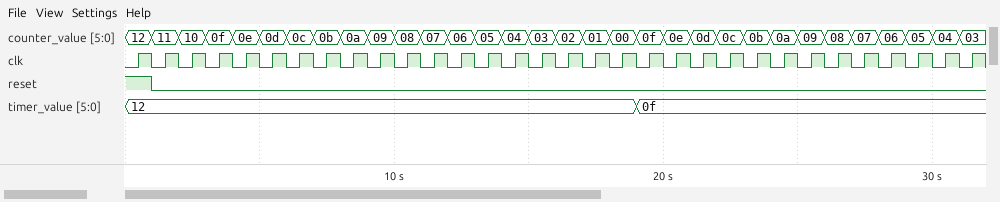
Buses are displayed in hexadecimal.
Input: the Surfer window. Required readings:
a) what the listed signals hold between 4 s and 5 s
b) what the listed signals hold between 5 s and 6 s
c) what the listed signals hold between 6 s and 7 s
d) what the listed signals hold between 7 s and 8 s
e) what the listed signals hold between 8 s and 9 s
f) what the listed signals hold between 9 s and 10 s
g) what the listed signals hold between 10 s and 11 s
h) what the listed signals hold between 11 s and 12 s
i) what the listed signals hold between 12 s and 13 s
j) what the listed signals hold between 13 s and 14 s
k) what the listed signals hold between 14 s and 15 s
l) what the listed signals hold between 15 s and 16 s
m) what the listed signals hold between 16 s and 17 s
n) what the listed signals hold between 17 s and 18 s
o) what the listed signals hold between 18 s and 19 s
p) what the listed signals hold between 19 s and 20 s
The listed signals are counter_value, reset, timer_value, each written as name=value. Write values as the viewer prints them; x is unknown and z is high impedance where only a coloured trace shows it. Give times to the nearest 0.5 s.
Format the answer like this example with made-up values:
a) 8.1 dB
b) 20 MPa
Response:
a) counter_value=0e, reset=0, timer_value=12
b) counter_value=0d, reset=0, timer_value=12
c) counter_value=0c, reset=0, timer_value=12
d) counter_value=0b, reset=0, timer_value=12
e) counter_value=0a, reset=0, timer_value=12
f) counter_value=09, reset=0, timer_value=12
g) counter_value=08, reset=0, timer_value=12
h) counter_value=07, reset=0, timer_value=12
i) counter_value=06, reset=0, timer_value=12
j) counter_value=05, reset=0, timer_value=12
k) counter_value=04, reset=0, timer_value=12
l) counter_value=03, reset=0, timer_value=12
m) counter_value=02, reset=0, timer_value=12
n) counter_value=01, reset=0, timer_value=12
o) counter_value=00, reset=0, timer_value=12
p) counter_value=0f, reset=0, timer_value=0f
